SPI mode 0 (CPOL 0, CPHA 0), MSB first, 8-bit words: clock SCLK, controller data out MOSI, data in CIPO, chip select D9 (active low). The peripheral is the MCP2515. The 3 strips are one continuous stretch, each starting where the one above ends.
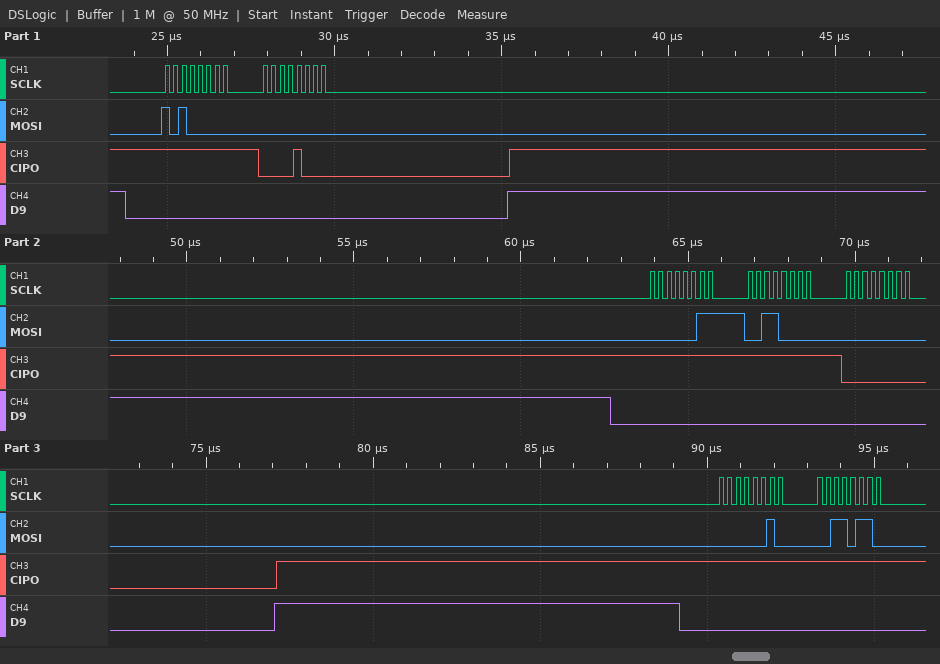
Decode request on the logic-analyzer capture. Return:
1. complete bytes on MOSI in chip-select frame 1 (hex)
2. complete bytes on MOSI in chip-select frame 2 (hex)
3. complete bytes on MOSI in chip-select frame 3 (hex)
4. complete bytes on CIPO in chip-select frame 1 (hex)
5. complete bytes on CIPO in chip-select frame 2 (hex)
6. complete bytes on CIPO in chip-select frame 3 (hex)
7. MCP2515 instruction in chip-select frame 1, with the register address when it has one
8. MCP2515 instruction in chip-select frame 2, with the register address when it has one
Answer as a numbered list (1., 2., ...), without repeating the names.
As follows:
1. A0 00
2. 03 30 00
3. 02 36
4. FF 08
5. FF FF 00
6. FF FF
7. READ STATUS
8. READ 0x30
